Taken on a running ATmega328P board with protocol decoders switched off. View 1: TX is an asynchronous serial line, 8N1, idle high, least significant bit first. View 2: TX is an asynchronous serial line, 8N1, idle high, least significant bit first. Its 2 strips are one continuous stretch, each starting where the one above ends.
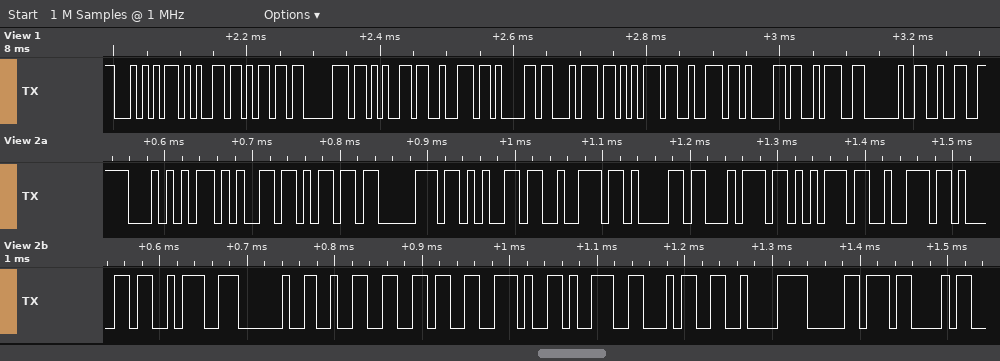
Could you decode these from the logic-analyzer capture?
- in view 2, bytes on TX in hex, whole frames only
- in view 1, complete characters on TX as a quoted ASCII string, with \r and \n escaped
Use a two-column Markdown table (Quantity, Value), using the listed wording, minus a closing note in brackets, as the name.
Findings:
| Quantity | Value |
|---|---|
| in view 2, bytes on TX in hex, whole frames only | 54 65 6D 70 65 72 61 74 75 72 61 3A 20 32 36 2E 39 34 C2 B0 43 |
| in view 1, complete characters on TX as a quoted ASCII string, with \r and \n escaped | "Temperatura: 2" |
